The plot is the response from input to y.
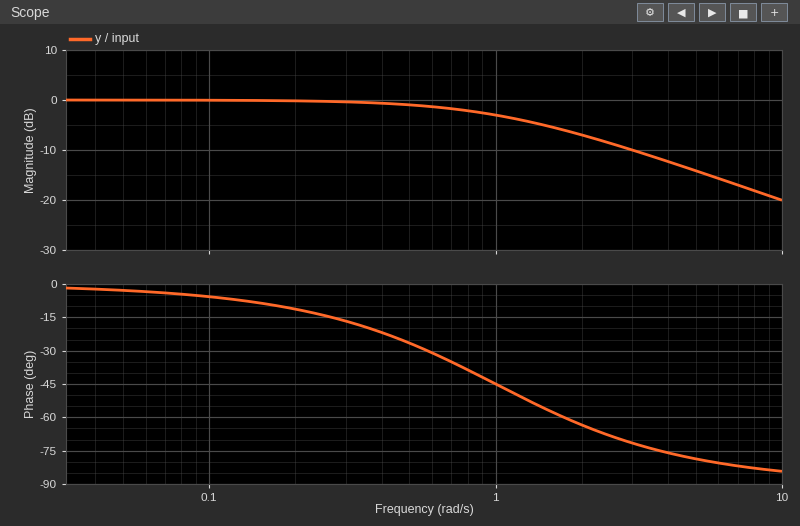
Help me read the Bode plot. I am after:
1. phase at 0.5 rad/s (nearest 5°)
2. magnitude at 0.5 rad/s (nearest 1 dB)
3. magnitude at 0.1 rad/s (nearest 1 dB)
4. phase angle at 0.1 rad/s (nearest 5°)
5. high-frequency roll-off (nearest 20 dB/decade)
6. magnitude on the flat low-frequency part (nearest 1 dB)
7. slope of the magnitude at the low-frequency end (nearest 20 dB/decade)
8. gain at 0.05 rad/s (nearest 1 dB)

-25°
-1 dB
0 dB
-5°
-20 dB/decade
0 dB
0 dB/decade
0 dB
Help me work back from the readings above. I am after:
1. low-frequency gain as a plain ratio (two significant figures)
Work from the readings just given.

1.0
